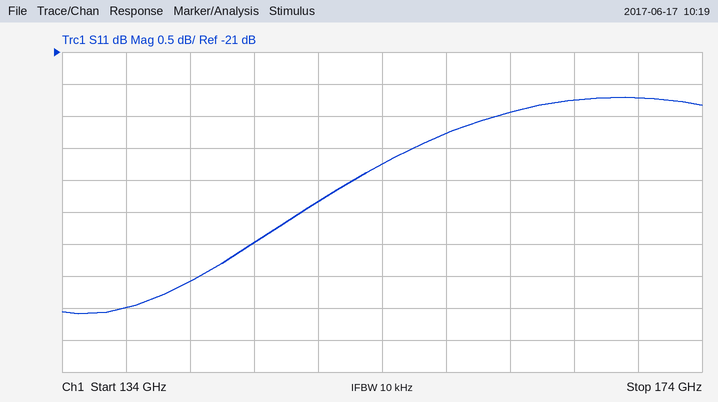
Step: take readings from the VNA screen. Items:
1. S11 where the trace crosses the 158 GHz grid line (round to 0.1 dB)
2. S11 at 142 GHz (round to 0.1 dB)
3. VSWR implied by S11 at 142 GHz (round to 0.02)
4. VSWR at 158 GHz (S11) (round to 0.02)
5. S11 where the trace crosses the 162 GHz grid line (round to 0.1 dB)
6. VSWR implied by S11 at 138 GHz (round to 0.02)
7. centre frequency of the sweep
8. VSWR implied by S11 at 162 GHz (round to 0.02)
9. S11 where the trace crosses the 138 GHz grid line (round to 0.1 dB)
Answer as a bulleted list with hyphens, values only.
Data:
- -22.3 dB
- -24.6 dB
- 1.12
- 1.16
- -21.9 dB
- 1.12
- 154 GHz
- 1.18
- -25.0 dB
